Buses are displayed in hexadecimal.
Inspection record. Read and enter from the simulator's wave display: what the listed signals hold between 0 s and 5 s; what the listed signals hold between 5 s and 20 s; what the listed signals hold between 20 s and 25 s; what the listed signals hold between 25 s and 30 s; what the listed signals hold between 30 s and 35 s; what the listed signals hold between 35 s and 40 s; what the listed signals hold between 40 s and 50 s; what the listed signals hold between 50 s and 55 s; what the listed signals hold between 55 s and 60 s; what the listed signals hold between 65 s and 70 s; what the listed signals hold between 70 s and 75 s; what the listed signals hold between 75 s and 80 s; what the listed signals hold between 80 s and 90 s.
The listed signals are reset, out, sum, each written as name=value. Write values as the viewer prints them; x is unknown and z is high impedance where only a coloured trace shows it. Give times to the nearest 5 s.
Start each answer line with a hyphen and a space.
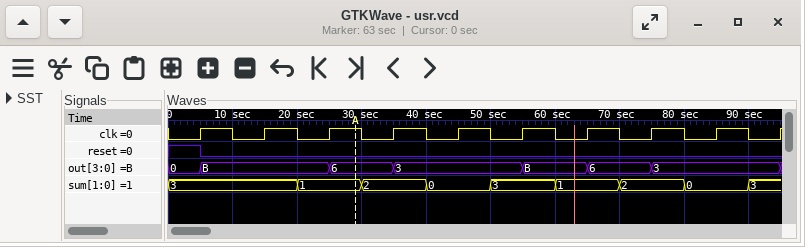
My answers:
- reset=1, out=0, sum=3
- reset=0, out=B, sum=3
- reset=0, out=B, sum=1
- reset=0, out=6, sum=1
- reset=0, out=6, sum=2
- reset=0, out=3, sum=2
- reset=0, out=3, sum=0
- reset=0, out=3, sum=3
- reset=0, out=B, sum=3
- reset=0, out=6, sum=1
- reset=0, out=6, sum=2
- reset=0, out=3, sum=2
- reset=0, out=3, sum=0
